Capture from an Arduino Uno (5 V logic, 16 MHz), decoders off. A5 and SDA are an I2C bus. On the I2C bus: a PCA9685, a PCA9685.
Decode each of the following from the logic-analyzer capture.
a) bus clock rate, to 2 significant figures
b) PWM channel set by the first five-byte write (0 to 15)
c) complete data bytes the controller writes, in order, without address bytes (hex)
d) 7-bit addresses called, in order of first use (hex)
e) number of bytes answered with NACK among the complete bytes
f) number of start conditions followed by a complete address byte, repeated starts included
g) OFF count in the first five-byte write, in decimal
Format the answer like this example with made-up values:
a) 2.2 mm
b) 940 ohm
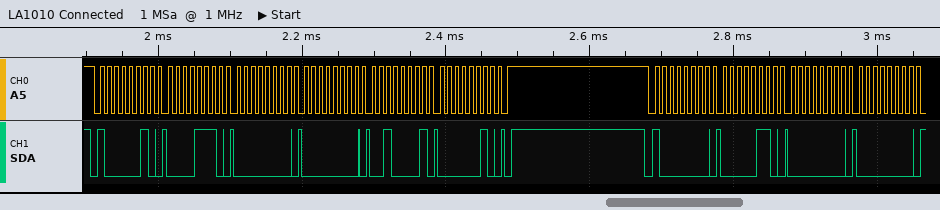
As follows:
a) 100 kHz
b) 2
c) 0E 00 00 21 02 06 00 00
d) 0x41 0x40
e) 0
f) 2
g) 545
